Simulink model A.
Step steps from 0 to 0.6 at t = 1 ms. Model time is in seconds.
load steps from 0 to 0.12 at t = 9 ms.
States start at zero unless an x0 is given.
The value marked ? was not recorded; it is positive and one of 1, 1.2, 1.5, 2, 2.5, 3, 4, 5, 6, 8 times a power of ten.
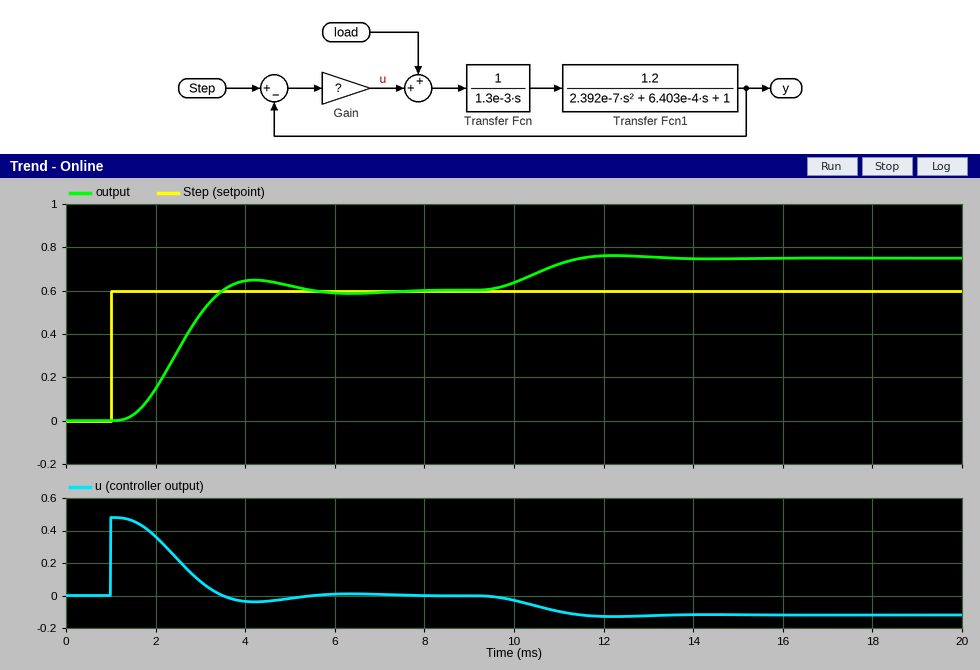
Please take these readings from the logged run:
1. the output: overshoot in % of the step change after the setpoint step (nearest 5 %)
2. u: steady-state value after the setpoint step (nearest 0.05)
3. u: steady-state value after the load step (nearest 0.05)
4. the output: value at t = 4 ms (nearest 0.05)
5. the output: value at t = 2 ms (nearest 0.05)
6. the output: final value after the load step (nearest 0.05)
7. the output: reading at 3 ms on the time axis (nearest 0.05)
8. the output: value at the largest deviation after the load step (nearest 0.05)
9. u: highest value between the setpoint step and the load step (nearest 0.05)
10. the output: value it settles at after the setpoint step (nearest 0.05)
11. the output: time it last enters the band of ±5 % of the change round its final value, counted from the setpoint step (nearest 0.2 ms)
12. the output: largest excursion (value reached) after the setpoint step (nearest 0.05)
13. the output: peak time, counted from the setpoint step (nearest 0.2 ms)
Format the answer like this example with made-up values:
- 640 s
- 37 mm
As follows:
- 10 %
- 0.00
- -0.10
- 0.65
- 0.15
- 0.75
- 0.50
- 0.75
- 0.50
- 0.60
- 3.8 ms
- 0.65
- 3.2 ms
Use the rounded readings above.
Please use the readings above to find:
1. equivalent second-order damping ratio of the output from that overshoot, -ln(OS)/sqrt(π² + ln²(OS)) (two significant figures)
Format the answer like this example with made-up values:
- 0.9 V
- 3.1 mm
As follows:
- 0.59
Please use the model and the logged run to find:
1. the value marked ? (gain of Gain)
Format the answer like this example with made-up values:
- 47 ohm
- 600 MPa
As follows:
- 0.8
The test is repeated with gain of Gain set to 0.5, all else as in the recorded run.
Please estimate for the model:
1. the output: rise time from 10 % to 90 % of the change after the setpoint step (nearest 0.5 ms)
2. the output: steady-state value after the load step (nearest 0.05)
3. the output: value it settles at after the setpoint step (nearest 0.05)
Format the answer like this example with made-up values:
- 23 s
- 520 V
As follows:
- 3.0 ms
- 0.85
- 0.60
